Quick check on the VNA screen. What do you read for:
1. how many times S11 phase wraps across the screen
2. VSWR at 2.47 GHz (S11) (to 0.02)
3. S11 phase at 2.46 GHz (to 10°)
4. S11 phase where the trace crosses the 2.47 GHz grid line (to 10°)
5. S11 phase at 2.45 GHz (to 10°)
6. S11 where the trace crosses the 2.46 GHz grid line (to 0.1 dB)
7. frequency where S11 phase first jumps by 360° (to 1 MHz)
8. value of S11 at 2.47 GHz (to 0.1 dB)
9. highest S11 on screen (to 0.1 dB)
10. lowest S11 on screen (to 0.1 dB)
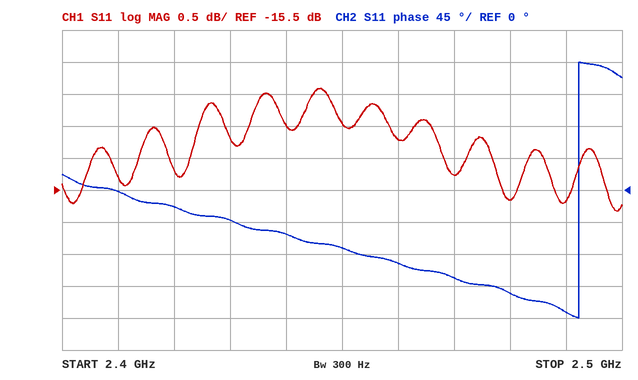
1
1.42
-100°
-120°
-80°
-14.7 dB
2.492 GHz
-15.3 dB
-13.9 dB
-15.8 dB
